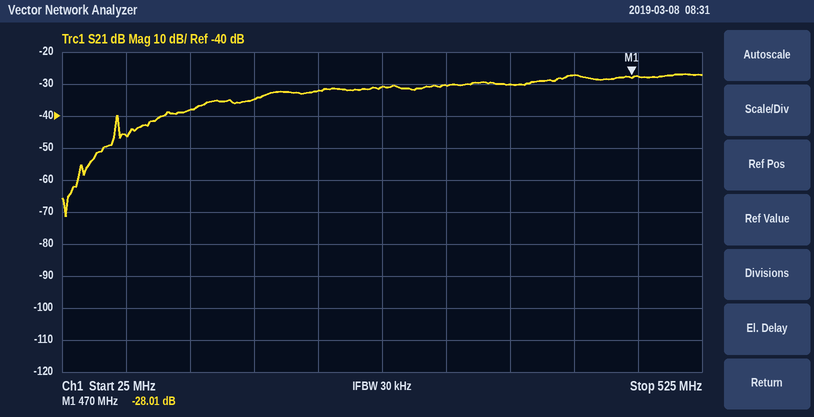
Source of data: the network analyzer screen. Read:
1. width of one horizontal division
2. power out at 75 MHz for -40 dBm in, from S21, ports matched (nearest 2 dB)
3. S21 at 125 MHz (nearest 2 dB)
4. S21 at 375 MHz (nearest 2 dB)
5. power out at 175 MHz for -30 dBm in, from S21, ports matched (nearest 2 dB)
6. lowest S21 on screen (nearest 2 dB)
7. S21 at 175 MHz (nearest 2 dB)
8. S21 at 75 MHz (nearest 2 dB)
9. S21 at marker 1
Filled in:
50 MHz
-86 dBm
-38 dB
-30 dB
-64 dBm
-72 dB
-34 dB
-46 dB
-28.01 dB
